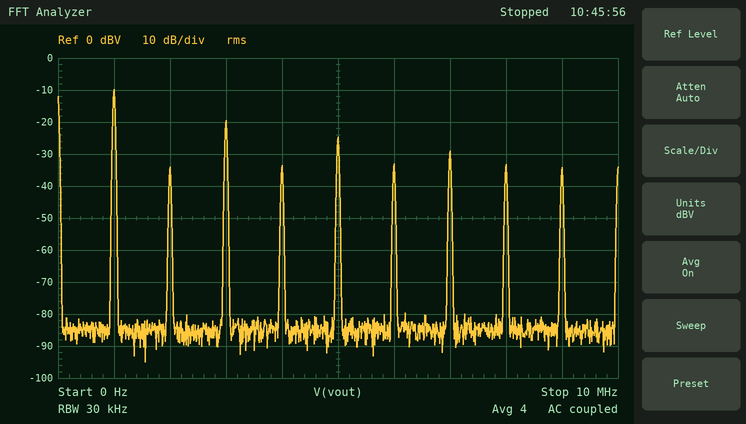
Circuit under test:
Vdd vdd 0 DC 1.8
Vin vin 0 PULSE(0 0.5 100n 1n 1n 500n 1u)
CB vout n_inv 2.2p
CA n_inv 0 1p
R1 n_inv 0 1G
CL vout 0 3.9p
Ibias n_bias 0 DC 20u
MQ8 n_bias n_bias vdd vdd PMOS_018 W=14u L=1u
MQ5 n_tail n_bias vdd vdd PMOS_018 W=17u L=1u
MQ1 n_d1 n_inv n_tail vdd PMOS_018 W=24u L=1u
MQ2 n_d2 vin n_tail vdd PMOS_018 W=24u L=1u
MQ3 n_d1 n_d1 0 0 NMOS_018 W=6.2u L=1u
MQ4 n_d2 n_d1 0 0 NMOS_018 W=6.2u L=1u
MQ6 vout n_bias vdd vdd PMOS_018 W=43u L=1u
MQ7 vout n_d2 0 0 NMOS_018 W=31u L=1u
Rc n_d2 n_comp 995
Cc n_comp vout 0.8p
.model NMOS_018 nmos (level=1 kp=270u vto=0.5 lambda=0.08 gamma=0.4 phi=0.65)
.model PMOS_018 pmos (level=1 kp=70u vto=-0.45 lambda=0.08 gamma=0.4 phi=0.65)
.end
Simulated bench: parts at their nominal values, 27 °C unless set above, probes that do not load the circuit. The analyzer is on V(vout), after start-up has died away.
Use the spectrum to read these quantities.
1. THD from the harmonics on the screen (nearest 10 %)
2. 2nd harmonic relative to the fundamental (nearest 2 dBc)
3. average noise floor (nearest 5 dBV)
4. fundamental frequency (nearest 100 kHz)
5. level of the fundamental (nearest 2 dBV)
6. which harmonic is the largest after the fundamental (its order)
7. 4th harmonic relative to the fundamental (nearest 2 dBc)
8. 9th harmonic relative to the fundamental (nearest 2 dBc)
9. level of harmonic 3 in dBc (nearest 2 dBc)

40 %
-24 dBc
-85 dBV
1.0 MHz
-10 dBV
3
-24 dBc
-24 dBc
-10 dBc
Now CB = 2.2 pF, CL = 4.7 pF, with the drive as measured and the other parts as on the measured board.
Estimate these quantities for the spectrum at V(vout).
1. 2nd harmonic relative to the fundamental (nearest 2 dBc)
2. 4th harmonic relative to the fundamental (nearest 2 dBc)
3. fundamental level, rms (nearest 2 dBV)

-22 dBc
-22 dBc
-10 dBV
